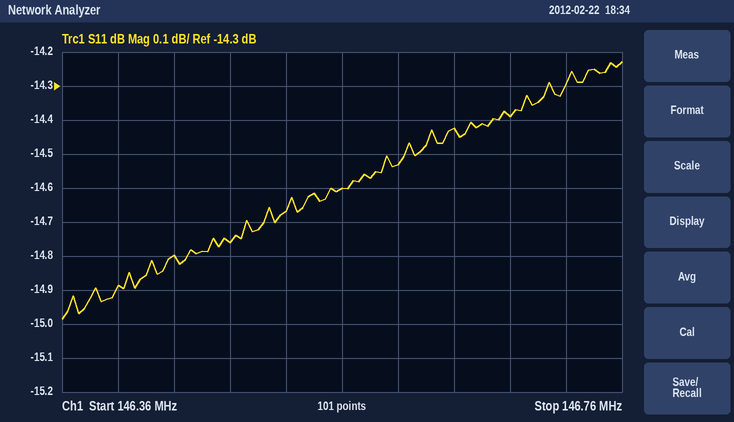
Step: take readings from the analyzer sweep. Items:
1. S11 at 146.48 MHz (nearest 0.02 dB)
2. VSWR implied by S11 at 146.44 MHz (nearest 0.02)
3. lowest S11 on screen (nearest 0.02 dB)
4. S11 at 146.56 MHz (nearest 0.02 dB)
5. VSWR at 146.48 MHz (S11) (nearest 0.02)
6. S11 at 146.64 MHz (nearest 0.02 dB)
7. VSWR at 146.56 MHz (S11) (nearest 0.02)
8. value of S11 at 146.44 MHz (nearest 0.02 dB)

-14.76 dB
1.44
-14.98 dB
-14.60 dB
1.44
-14.42 dB
1.46
-14.80 dB
